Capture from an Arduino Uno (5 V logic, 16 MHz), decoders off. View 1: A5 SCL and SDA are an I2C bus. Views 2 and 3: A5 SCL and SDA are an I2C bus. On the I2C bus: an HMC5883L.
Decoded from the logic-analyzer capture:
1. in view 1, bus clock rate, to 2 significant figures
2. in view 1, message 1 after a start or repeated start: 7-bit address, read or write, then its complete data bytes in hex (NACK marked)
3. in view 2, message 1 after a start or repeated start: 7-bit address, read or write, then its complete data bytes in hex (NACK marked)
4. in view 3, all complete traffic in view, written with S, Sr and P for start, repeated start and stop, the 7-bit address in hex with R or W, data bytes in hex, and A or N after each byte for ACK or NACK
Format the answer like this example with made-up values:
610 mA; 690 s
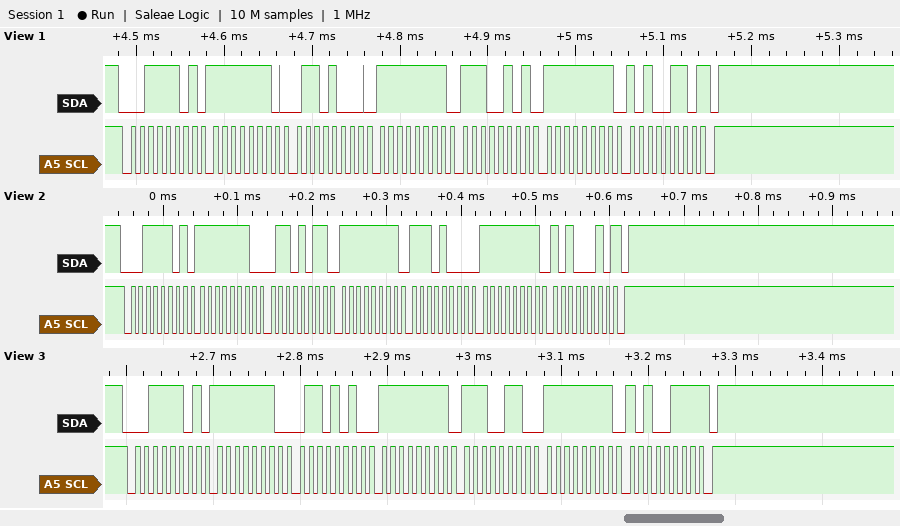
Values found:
100 kHz; 0x1E read: FE 68 FF E5 FF A6 NACK; 0x1E read: FE 6B FF E8 FF A2 NACK; S 1ER A FE A 6A A FF A E6 A FF A A7 N P
